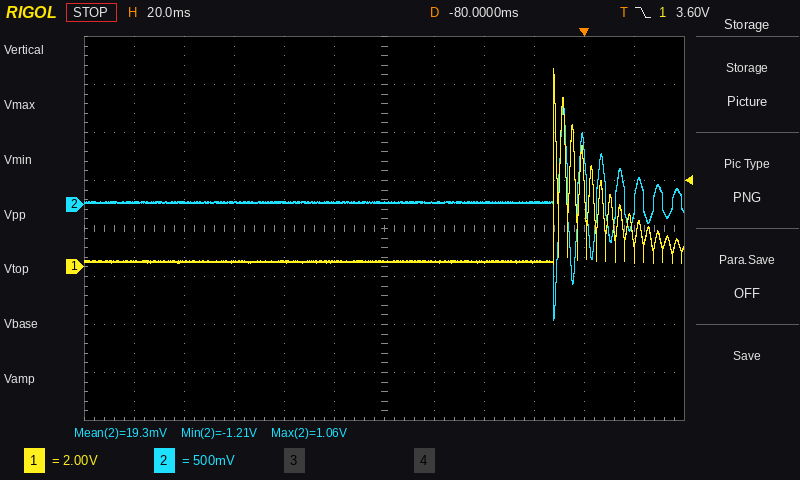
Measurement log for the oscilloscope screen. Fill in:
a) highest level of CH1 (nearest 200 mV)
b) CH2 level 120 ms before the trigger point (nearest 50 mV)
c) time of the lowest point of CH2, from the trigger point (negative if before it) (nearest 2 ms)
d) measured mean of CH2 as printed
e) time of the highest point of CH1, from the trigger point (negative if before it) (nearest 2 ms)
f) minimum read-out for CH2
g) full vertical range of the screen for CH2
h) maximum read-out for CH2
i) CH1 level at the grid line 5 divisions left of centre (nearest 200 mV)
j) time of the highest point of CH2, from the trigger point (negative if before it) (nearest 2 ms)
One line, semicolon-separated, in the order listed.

8.2 V; 0 mV; -12 ms; 19.3 mV; -12 ms; -1.21 V; 4 V; 1.06 V; 200 mV; -8 ms
